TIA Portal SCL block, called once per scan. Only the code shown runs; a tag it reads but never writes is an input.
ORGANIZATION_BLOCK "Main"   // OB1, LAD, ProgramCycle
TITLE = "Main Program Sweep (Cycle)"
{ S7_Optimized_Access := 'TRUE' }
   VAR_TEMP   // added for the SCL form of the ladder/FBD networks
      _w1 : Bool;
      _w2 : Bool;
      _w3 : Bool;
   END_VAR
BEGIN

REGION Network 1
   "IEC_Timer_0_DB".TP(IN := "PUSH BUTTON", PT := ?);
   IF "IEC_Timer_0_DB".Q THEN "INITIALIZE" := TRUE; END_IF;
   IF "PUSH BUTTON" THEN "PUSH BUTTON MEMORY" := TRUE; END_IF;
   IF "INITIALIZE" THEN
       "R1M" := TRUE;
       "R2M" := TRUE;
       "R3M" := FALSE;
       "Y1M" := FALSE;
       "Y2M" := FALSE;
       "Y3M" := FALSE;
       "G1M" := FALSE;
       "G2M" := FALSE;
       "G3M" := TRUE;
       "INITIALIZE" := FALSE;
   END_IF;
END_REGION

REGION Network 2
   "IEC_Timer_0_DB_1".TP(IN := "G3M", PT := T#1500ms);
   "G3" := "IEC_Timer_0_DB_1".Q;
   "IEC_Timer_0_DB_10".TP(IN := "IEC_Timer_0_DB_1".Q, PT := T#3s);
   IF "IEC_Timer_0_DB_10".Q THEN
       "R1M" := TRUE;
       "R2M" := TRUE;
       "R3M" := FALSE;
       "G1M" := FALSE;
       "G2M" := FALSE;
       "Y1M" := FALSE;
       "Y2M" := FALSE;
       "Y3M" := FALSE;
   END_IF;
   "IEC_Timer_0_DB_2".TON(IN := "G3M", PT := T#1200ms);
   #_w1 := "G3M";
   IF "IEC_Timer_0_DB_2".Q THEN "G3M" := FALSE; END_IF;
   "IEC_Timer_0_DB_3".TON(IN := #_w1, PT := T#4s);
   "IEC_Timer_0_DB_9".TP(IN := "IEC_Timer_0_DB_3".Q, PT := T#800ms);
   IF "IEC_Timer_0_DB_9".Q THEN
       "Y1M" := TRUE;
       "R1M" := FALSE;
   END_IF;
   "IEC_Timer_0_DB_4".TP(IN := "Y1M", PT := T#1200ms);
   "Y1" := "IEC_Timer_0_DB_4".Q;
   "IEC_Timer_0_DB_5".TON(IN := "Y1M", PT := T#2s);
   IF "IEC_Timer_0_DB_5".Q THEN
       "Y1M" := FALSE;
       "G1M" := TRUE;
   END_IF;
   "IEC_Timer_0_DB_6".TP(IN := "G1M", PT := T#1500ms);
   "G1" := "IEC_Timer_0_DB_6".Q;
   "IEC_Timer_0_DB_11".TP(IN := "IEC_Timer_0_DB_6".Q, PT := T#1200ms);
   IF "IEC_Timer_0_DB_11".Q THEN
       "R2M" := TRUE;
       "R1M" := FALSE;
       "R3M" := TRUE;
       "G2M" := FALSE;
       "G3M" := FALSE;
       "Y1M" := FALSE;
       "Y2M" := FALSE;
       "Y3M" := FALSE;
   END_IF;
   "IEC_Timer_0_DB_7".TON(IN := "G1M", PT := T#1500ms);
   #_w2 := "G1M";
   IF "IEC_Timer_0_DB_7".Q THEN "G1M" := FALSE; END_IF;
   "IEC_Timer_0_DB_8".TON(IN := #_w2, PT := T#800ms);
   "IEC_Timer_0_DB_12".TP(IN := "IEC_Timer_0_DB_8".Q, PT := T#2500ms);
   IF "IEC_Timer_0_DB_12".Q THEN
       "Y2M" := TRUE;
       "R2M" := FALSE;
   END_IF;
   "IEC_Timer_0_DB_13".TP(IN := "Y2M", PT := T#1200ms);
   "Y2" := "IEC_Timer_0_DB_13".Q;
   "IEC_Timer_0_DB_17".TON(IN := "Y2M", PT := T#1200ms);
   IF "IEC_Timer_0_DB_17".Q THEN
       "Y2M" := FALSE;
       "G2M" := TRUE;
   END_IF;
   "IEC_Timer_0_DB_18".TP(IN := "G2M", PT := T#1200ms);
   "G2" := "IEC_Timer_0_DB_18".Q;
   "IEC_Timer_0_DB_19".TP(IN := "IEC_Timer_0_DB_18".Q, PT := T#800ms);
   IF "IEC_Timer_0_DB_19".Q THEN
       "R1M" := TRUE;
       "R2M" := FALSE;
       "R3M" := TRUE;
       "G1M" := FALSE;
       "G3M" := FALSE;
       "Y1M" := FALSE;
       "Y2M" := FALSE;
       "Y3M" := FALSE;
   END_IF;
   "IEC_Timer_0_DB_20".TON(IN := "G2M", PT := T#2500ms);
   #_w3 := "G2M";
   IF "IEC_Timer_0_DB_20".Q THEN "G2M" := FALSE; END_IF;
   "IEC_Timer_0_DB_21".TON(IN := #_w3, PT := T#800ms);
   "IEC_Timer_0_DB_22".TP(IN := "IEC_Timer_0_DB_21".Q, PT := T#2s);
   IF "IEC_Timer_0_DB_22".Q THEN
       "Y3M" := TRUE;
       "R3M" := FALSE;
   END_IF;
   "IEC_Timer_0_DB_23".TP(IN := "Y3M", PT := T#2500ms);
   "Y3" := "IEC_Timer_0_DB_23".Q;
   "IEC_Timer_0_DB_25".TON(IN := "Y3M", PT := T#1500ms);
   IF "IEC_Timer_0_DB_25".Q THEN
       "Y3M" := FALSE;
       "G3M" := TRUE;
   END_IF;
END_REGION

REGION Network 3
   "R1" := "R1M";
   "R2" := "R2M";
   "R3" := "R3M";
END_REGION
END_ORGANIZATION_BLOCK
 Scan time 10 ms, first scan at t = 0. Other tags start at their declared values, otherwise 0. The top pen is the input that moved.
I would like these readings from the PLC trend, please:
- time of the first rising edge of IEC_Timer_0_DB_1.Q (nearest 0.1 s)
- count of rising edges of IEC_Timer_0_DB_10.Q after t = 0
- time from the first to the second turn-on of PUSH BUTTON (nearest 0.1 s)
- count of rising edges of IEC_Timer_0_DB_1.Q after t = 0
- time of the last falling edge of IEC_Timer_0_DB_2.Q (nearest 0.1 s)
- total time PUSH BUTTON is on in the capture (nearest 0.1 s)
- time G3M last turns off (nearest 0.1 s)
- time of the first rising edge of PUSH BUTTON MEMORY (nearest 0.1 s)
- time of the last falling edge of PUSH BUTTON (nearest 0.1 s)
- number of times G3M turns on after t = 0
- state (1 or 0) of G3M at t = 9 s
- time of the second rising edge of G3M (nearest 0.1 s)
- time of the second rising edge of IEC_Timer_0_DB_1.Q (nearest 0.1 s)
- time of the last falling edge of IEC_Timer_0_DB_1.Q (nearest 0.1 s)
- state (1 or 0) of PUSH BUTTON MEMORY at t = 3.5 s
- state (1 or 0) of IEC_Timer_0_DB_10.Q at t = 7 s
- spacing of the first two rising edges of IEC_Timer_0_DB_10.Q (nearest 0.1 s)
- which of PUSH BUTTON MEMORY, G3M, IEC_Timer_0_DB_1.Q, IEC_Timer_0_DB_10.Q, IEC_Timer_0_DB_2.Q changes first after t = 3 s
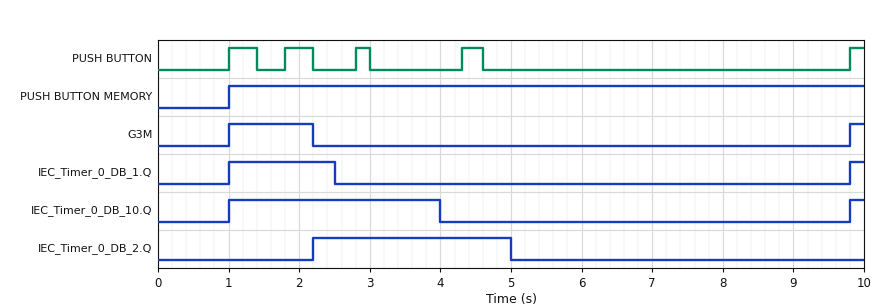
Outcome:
1.0 s
2
0.8 s
2
5.0 s
1.5 s
2.2 s
1.0 s
4.6 s
2
0
9.8 s
9.8 s
2.5 s
1
0
8.8 s
IEC_Timer_0_DB_10.Q
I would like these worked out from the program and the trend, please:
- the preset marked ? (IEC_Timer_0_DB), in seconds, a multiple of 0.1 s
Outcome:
4.0 s
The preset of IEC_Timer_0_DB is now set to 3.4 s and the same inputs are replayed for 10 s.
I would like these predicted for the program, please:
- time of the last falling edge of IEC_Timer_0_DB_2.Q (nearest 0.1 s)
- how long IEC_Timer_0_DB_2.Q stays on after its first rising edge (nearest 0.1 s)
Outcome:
4.4 s
2.2 s
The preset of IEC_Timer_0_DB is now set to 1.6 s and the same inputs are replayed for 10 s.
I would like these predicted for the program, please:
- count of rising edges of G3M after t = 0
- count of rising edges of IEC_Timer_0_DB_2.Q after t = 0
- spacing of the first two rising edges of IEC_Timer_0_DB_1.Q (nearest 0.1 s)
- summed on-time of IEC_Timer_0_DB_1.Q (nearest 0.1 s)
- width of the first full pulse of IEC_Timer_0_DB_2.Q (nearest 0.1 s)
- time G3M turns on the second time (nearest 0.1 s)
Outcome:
3
2
1.8 s
3.2 s
0.4 s
2.8 s
